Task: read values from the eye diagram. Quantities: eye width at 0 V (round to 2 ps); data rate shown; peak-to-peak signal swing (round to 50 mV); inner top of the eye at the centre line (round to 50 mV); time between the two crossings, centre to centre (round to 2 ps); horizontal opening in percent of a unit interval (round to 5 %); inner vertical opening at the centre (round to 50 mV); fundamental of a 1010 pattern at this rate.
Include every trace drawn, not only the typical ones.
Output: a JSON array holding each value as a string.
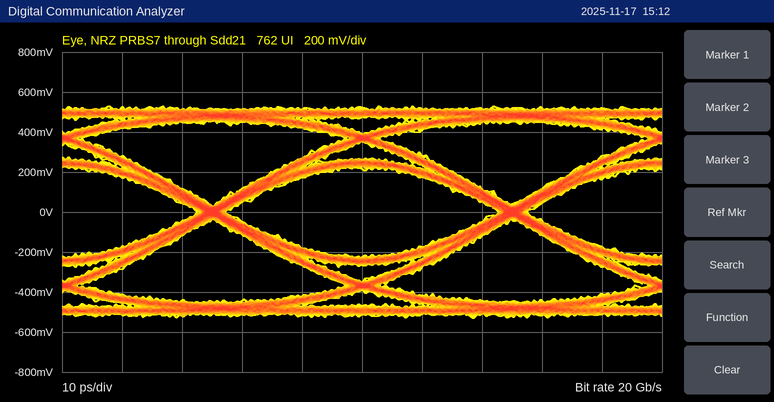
["46 ps", "20 Gb/s", "1.05 V", "200 mV", "50 ps", "90 %", "450 mV", "10 GHz"]
